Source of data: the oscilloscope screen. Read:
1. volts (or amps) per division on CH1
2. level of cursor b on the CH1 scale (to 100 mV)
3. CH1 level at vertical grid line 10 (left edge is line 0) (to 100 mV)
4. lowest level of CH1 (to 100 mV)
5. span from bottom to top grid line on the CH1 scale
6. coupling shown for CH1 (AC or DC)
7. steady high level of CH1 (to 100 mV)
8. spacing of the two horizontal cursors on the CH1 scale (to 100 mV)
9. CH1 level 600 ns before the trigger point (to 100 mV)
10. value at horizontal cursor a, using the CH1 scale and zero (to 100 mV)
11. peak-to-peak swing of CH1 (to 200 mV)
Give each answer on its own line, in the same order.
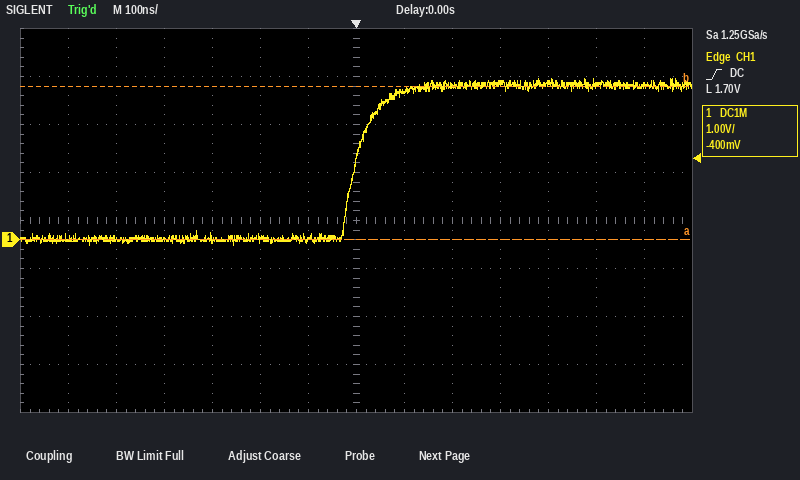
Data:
1 V
3.2 V
3.3 V
-100 mV
8 V
DC
3.2 V
3.2 V
0.0 V
0.0 V
3.4 V
